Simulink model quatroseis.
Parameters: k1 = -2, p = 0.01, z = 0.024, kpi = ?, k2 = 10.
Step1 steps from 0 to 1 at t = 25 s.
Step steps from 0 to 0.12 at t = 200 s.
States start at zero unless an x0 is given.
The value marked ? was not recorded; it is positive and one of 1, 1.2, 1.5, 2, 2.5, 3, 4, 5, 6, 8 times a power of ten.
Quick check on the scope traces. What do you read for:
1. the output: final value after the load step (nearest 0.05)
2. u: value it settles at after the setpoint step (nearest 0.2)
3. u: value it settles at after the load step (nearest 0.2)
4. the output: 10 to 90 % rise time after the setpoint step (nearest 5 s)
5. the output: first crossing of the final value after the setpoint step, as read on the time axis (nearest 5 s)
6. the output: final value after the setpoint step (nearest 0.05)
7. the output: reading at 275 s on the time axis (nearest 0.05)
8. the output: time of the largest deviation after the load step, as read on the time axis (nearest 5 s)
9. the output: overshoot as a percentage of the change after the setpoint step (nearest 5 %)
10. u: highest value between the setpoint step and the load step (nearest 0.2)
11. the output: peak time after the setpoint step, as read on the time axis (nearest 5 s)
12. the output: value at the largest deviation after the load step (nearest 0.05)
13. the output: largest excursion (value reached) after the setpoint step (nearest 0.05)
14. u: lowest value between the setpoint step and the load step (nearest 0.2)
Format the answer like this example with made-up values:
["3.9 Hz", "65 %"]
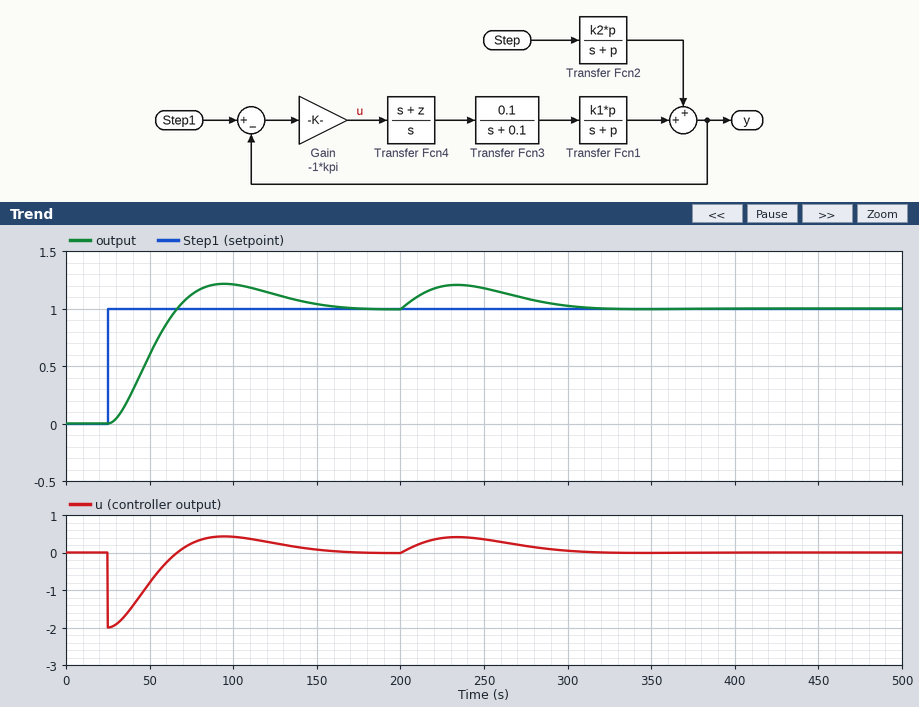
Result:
["1.00", "0.0", "0.0", "30 s", "65 s", "1.00", "1.10", "235 s", "20 %", "0.4", "95 s", "1.20", "1.20", "-2.0"]
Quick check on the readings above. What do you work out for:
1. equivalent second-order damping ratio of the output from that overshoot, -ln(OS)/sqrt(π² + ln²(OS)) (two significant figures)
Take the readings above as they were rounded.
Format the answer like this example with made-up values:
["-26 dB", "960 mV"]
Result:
["0.46"]
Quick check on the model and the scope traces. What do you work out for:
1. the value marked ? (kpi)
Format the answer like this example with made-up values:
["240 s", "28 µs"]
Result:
["2"]
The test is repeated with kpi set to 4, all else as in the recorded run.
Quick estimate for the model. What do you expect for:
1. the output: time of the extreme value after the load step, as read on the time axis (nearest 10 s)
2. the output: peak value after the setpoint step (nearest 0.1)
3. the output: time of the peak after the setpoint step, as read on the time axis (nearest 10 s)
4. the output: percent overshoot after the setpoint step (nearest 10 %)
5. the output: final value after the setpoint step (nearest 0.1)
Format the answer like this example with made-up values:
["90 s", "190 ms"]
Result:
["220 s", "1.3", "70 s", "30 %", "1.0"]
